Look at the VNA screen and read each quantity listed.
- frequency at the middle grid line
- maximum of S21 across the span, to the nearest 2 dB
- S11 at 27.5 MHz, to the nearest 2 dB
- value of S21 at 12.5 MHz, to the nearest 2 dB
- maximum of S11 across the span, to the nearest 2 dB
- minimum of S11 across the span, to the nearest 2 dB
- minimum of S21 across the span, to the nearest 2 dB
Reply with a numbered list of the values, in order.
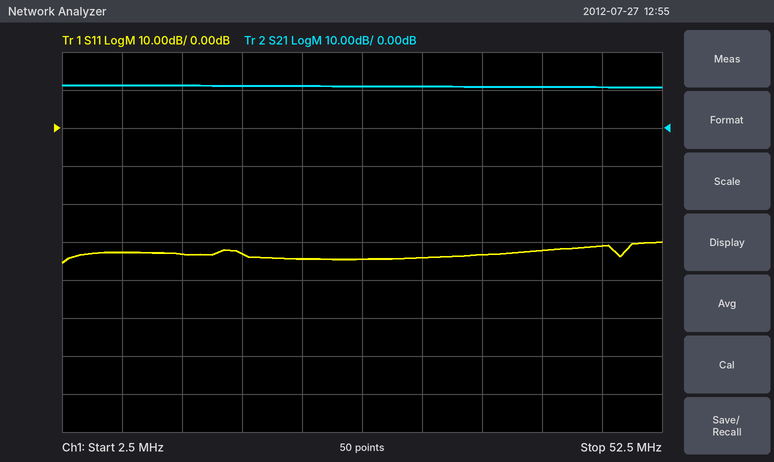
1. 27.5 MHz
2. 12 dB
3. -34 dB
4. 12 dB
5. -30 dB
6. -36 dB
7. 10 dB
